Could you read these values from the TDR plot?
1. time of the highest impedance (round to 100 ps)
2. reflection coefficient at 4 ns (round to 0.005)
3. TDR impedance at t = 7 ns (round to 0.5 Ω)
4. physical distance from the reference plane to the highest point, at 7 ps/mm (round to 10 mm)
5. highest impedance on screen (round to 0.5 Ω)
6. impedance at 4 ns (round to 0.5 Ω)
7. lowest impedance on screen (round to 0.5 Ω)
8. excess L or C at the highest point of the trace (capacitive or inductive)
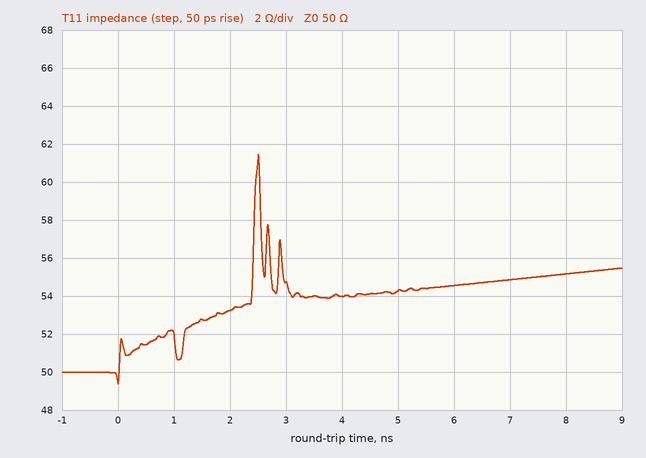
2.5 ns
+0.040
55.0 Ω
180 mm
61.5 Ω
54.0 Ω
49.5 Ω
inductive
